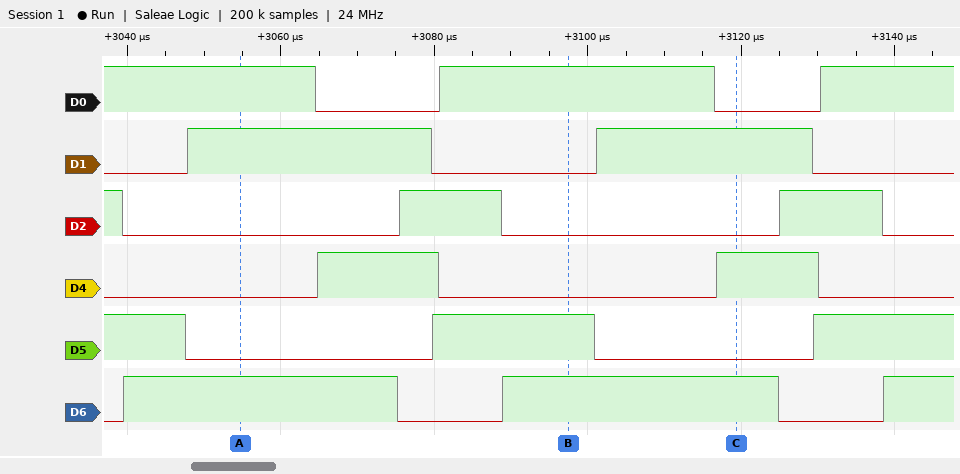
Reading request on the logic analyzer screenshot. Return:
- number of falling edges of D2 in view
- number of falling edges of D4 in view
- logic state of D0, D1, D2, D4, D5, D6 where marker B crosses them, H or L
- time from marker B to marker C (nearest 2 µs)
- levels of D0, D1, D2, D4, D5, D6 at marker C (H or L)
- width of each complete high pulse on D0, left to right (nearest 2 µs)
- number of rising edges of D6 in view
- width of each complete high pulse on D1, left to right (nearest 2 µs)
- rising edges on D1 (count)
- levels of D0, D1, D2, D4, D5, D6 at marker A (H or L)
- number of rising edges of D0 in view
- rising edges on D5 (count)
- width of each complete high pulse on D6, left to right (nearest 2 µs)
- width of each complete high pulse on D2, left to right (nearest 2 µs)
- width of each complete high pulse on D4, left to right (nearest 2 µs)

3
2
D0=H, D1=L, D2=L, D4=L, D5=H, D6=H
22 µs
D0=L, D1=H, D2=L, D4=H, D5=L, D6=H
36 µs
3
32 µs, 28 µs
2
D0=H, D1=H, D2=L, D4=L, D5=L, D6=H
2
2
36 µs, 36 µs
14 µs, 14 µs
16 µs, 14 µs
